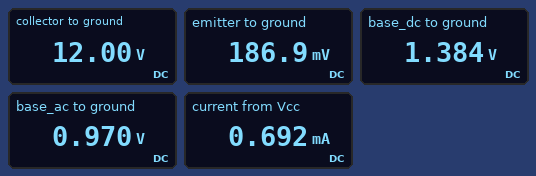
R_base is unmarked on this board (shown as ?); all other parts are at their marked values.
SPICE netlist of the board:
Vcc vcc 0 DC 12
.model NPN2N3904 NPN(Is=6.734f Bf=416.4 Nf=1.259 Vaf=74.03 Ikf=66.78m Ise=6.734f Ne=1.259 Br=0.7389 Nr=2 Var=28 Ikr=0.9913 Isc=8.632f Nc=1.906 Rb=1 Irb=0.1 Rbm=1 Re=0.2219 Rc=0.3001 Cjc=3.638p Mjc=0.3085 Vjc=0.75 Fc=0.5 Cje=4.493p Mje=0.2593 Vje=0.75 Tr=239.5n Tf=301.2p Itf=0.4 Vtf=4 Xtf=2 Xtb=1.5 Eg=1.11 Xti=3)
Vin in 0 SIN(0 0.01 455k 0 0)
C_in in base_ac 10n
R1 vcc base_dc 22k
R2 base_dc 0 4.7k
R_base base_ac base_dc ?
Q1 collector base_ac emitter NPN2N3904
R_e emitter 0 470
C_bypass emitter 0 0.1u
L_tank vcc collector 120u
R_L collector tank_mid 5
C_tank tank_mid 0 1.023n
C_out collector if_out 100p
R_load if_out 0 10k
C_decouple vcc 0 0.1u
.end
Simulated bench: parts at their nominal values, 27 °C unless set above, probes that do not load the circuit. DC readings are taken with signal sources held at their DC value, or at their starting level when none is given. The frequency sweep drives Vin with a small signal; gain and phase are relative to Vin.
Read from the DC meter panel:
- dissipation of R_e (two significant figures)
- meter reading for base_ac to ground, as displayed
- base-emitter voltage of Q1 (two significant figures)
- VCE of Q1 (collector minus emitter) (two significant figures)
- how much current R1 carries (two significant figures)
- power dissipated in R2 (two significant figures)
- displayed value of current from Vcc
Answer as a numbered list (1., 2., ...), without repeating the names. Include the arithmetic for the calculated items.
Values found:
1. (186.9 mV)^2 / 470 Ω = 74 µW
2. 0.970 V
3. 970 mV - 186.9 mV = 780 mV
4. 12 V - 186.9 mV = 12 V
5. (12 V - 1.384 V) / 22 kΩ = 480 µA
6. (1.384 V)^2 / 4.7 kΩ = 410 µW
7. 0.692 mA
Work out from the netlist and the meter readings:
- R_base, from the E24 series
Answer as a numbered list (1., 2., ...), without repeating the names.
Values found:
1. 2.2 kΩ
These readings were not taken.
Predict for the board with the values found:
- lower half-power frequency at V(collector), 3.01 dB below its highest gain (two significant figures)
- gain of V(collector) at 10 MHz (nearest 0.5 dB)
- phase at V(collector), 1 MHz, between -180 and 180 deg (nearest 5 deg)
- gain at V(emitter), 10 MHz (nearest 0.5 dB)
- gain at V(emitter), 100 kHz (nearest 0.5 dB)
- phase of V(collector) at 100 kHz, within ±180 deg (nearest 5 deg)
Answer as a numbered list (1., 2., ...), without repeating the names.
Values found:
1. 440 kHz
2. -19.5 dB
3. 100 deg
4. -54.5 dB
5. -18.0 dB
6. -40 deg
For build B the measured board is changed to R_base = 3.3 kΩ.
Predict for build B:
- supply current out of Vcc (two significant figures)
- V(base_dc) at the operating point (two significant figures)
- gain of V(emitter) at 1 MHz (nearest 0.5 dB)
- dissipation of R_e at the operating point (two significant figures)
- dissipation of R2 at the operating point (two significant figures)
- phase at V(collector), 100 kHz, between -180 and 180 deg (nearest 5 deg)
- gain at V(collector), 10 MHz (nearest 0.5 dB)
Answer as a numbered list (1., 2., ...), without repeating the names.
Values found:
1. 660 µA
2. 1.5 V
3. -35.5 dB
4. 56 µW
5. 470 µW
6. -45 deg
7. -21.0 dB
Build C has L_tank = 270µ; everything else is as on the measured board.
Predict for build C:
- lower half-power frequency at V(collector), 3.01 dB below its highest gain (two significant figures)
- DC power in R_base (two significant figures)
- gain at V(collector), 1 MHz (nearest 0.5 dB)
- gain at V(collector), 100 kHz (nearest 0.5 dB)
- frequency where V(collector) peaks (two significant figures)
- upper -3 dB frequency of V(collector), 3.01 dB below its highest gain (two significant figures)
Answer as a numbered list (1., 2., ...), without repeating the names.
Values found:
1. 290 kHz
2. 78 µW
3. 0.5 dB
4. -2.0 dB
5. 300 kHz
6. 310 kHz
